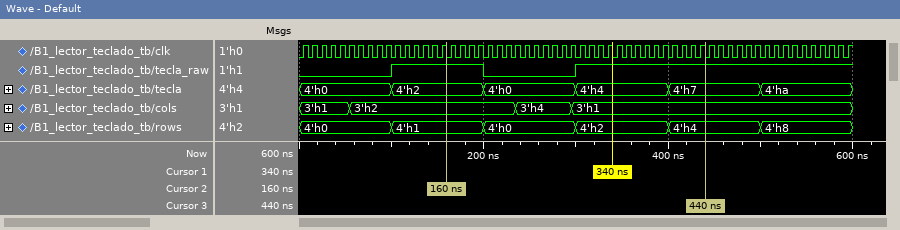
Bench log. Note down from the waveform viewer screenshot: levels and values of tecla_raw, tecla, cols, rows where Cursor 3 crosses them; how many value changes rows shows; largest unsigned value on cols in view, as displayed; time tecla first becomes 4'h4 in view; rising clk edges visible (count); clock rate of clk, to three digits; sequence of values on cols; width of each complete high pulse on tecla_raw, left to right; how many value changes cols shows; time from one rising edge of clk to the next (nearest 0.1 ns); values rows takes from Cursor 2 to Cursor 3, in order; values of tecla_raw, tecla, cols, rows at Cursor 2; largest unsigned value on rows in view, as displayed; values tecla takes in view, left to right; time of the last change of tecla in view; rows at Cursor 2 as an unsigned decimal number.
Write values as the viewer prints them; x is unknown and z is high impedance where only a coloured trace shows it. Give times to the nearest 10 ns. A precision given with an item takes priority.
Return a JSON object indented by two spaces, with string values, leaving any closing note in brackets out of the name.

{
  "levels and values of tecla_raw, tecla, cols, rows where Cursor 3 crosses them": "tecla_raw=1, tecla=4'h7, cols=3'h1, rows=4'h4",
  "how many value changes rows shows": "5",
  "largest unsigned value on cols in view, as displayed": "3'h4",
  "time tecla first becomes 4'h4 in view": "300 ns",
  "rising clk edges visible": "60",
  "clock rate of clk, to three digits": "100 MHz",
  "sequence of values on cols": "3'h1, 3'h2, 3'h4, 3'h1",
  "width of each complete high pulse on tecla_raw, left to right": "100 ns",
  "how many value changes cols shows": "3",
  "time from one rising edge of clk to the next": "10 ns",
  "values rows takes from Cursor 2 to Cursor 3, in order": "4'h1, 4'h0, 4'h2, 4'h4",
  "values of tecla_raw, tecla, cols, rows at Cursor 2": "tecla_raw=1, tecla=4'h2, cols=3'h2, rows=4'h1",
  "largest unsigned value on rows in view, as displayed": "4'h8",
  "values tecla takes in view, left to right": "4'h0, 4'h2, 4'h0, 4'h4, 4'h7, 4'ha",
  "time of the last change of tecla in view": "500 ns",
  "rows at Cursor 2 as an unsigned decimal number": "1"
}
